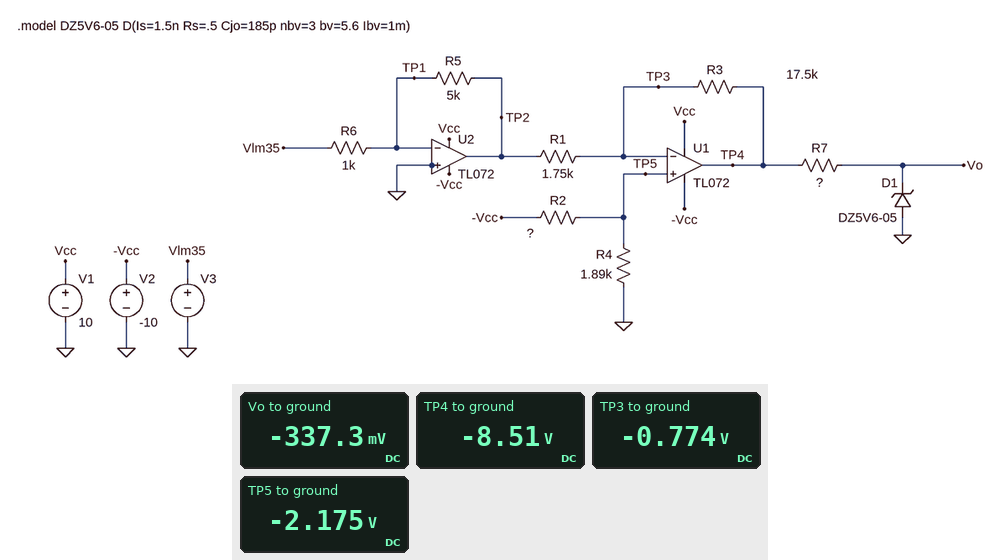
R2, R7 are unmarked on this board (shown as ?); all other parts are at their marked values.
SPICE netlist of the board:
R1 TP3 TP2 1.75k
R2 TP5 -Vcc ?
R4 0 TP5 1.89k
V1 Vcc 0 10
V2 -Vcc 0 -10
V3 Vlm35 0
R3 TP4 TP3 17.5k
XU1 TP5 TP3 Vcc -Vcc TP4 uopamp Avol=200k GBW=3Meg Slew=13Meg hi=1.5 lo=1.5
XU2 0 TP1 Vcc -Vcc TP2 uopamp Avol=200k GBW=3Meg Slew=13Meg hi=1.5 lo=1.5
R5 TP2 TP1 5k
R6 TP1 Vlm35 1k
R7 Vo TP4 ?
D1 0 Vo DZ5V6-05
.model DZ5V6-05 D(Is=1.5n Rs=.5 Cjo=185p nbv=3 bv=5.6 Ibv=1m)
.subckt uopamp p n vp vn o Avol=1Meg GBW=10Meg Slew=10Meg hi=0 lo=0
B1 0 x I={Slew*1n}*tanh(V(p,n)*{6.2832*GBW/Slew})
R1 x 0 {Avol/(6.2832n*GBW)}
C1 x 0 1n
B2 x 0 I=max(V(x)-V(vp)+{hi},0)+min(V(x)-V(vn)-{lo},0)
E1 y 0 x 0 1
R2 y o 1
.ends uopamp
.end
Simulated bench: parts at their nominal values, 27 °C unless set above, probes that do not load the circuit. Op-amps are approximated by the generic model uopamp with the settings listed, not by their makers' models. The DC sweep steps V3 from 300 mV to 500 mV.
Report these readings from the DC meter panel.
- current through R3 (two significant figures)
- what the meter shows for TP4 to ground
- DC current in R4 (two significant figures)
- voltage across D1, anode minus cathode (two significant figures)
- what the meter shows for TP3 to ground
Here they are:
440 µA
-8.51 V
1.2 mA
340 mV
-0.774 V
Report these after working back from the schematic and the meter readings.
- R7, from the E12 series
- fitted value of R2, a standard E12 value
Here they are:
12 kΩ
6.8 kΩ
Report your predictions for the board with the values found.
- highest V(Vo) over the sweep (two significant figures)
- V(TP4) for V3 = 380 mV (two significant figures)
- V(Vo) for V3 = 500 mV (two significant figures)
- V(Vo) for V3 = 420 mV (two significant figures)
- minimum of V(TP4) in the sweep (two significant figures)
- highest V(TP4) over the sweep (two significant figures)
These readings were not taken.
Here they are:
1.1 V
-4.9 V
1.1 V
-310 mV
-8.5 V
1.1 V
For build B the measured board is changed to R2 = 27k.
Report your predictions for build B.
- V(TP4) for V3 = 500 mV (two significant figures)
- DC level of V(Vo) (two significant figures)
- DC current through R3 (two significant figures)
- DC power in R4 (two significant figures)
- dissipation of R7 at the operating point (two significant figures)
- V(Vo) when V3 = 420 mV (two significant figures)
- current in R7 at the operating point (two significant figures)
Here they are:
8.5 V
-330 mV
370 µA
230 µW
3.9 mW
5.5 V
570 µA
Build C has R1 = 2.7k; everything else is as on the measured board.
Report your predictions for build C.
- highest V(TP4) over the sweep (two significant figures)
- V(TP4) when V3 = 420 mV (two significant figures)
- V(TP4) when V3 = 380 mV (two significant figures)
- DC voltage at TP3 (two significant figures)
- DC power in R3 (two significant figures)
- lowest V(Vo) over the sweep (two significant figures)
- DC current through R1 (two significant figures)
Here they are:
-68 mV
-2.7 V
-4.0 V
-1.1 V
3.1 mW
-330 mV
420 µA
